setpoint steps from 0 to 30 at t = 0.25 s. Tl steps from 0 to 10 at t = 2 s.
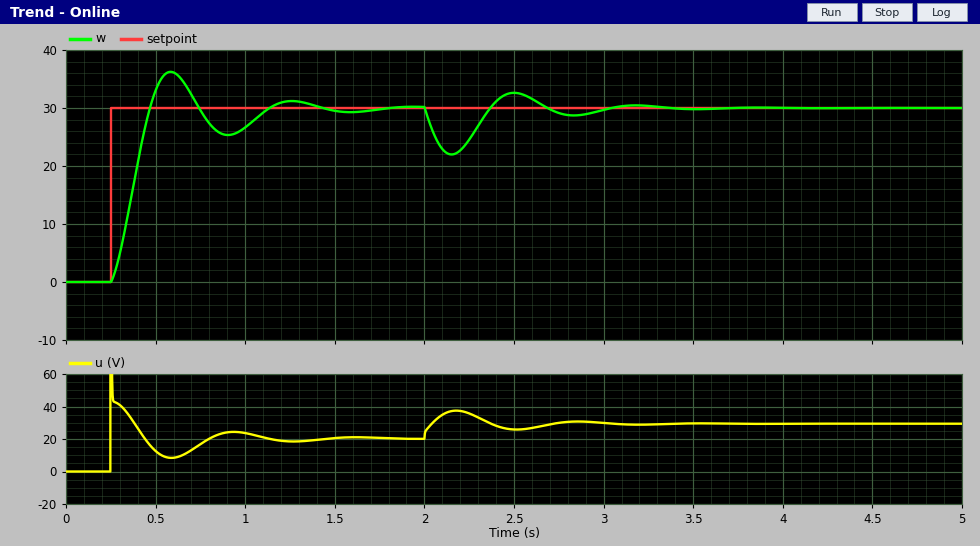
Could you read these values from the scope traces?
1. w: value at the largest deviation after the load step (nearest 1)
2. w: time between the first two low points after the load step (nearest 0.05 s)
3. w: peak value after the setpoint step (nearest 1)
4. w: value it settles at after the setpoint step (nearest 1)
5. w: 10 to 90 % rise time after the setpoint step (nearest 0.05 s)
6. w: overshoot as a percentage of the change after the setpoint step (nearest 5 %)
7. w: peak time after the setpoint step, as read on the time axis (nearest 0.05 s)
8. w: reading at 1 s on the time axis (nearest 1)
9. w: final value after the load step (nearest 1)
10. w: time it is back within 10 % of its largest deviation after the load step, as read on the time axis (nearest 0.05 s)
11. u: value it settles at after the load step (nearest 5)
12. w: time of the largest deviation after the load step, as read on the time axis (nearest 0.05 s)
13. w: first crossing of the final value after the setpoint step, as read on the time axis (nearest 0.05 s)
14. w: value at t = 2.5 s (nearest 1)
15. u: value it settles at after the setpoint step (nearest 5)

22
0.70 s
36
30
0.15 s
20 %
0.60 s
27
30
2.95 s
30
2.15 s
0.45 s
33
20
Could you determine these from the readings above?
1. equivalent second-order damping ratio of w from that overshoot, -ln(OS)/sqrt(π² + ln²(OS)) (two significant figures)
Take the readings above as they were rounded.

0.46
